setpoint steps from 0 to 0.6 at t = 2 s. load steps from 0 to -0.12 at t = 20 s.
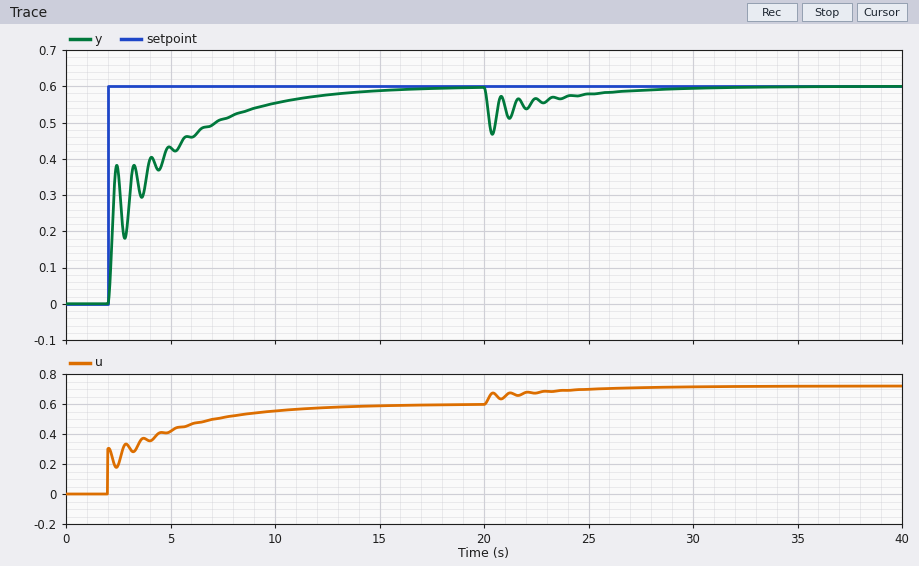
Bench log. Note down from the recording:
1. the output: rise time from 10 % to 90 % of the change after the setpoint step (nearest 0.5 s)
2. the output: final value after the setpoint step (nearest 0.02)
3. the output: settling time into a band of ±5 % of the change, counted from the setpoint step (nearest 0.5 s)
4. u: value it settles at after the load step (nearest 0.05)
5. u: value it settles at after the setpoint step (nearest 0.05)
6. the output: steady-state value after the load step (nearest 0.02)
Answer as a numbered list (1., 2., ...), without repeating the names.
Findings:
1. 7.0 s
2. 0.60
3. 9.5 s
4. 0.70
5. 0.60
6. 0.60
